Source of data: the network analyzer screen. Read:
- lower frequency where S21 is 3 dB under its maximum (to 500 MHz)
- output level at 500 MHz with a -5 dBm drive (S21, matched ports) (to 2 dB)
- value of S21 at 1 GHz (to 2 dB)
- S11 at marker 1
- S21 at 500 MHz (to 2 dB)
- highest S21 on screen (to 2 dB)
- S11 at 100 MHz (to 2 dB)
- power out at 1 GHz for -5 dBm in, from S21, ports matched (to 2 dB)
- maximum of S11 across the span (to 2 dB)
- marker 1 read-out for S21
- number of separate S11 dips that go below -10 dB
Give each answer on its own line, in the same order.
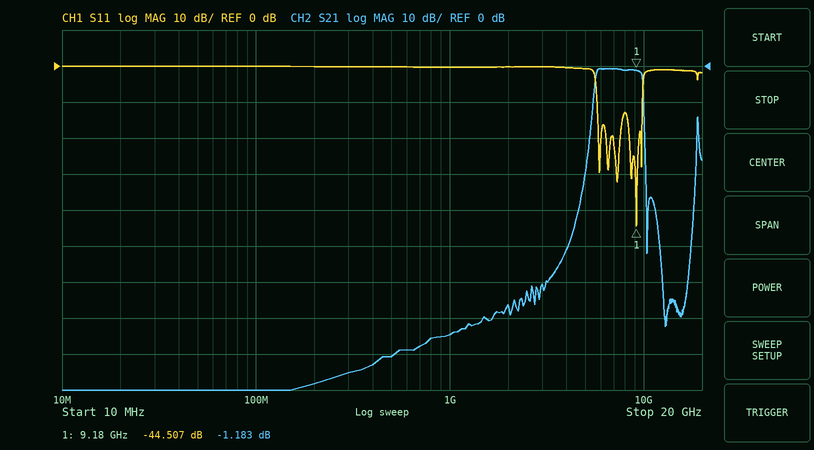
5.5 GHz
-86 dBm
-74 dB
-44.507 dB
-80 dB
0 dB
0 dB
-80 dBm
0 dB
-1.183 dB
6
